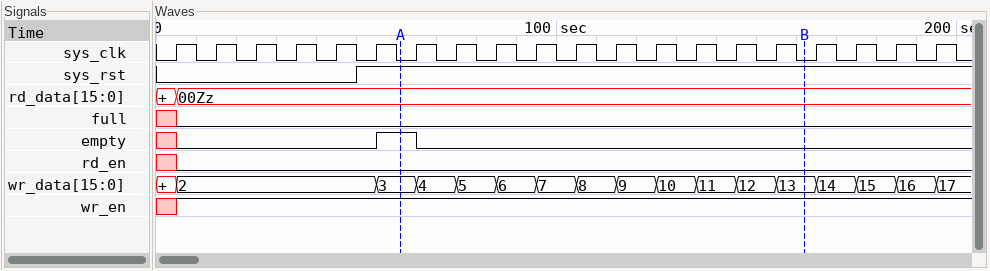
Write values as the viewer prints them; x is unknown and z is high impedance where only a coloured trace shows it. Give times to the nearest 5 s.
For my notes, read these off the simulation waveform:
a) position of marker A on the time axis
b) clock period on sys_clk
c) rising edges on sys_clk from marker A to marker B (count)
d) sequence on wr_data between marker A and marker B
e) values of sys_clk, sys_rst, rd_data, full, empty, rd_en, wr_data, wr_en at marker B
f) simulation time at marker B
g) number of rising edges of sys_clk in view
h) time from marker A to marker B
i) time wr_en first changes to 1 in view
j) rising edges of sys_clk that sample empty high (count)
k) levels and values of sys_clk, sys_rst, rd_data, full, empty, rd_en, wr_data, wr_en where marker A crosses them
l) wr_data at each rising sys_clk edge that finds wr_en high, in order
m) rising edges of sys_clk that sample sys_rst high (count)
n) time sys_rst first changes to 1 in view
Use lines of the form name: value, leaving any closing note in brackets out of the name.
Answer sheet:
position of marker A on the time axis: 60 s
clock period on sys_clk: 10 s
rising edges on sys_clk from marker A to marker B: 10
sequence on wr_data between marker A and marker B: 3, 4, 5, 6, 7, 8, 9, 10, 11, 12, 13
values of sys_clk, sys_rst, rd_data, full, empty, rd_en, wr_data, wr_en at marker B: sys_clk=0, sys_rst=1, rd_data=00Zz, full=0, empty=0, rd_en=0, wr_data=13, wr_en=1
simulation time at marker B: 160 s
number of rising edges of sys_clk in view: 20
time from marker A to marker B: 100 s
time wr_en first changes to 1 in view: 5 s
rising edges of sys_clk that sample empty high: 1
levels and values of sys_clk, sys_rst, rd_data, full, empty, rd_en, wr_data, wr_en where marker A crosses them: sys_clk=0, sys_rst=1, rd_data=00Zz, full=0, empty=1, rd_en=0, wr_data=3, wr_en=1
wr_data at each rising sys_clk edge that finds wr_en high, in order: 2, 2, 2, 2, 2, 3, 4, 5, 6, 7, 8, 9, 10, 11, 12, 13, 14, 15, 16
rising edges of sys_clk that sample sys_rst high: 15
time sys_rst first changes to 1 in view: 50 s
